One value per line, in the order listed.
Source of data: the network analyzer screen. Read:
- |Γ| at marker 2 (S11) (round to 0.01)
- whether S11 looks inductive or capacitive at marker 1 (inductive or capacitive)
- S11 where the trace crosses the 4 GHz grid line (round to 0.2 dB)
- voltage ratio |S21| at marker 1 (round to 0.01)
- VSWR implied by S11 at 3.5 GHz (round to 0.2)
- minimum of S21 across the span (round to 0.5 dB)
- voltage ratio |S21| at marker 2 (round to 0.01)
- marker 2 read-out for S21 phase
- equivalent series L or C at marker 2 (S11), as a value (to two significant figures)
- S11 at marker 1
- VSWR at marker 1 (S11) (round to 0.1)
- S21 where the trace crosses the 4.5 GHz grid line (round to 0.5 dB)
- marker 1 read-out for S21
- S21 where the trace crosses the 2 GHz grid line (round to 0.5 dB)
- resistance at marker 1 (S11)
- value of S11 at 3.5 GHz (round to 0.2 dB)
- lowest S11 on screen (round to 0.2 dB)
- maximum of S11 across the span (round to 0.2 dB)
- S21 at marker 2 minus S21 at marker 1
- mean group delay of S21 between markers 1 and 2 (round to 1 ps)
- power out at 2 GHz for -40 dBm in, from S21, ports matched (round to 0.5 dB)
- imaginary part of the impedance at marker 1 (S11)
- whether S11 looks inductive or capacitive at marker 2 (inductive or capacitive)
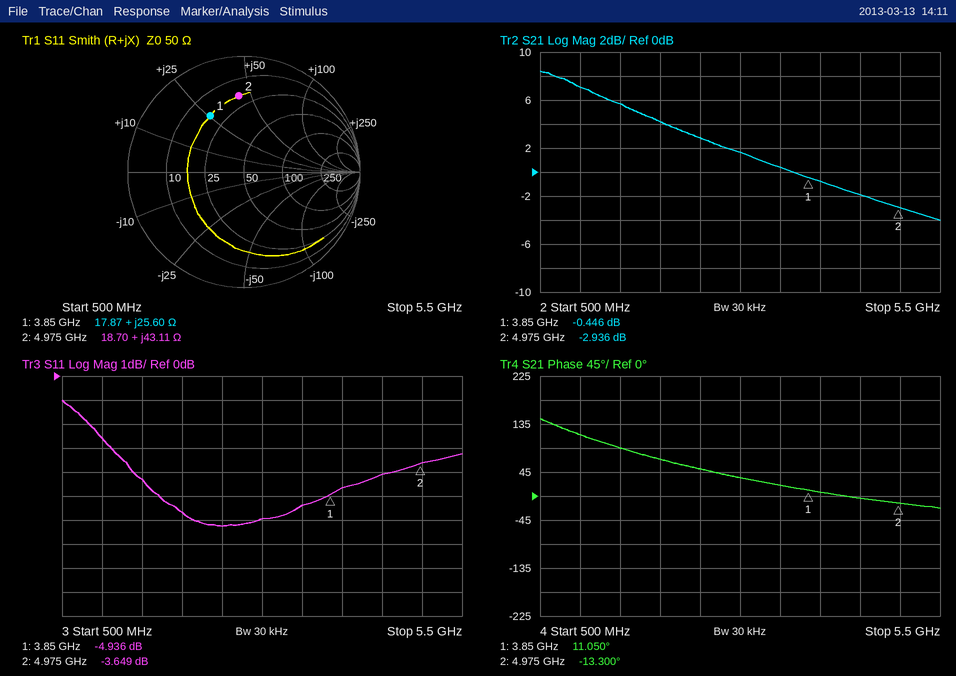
0.66
inductive
-4.6 dB
0.95
3.4
-4.0 dB
0.71
-13.300°
1.4 nH
-4.936 dB
3.6
-2.0 dB
-0.446 dB
4.0 dB
17.87 Ω
-5.4 dB
-6.2 dB
-1.0 dB
-2.490 dB
60 ps
-36.0 dBm
+25.60 Ω
inductive
